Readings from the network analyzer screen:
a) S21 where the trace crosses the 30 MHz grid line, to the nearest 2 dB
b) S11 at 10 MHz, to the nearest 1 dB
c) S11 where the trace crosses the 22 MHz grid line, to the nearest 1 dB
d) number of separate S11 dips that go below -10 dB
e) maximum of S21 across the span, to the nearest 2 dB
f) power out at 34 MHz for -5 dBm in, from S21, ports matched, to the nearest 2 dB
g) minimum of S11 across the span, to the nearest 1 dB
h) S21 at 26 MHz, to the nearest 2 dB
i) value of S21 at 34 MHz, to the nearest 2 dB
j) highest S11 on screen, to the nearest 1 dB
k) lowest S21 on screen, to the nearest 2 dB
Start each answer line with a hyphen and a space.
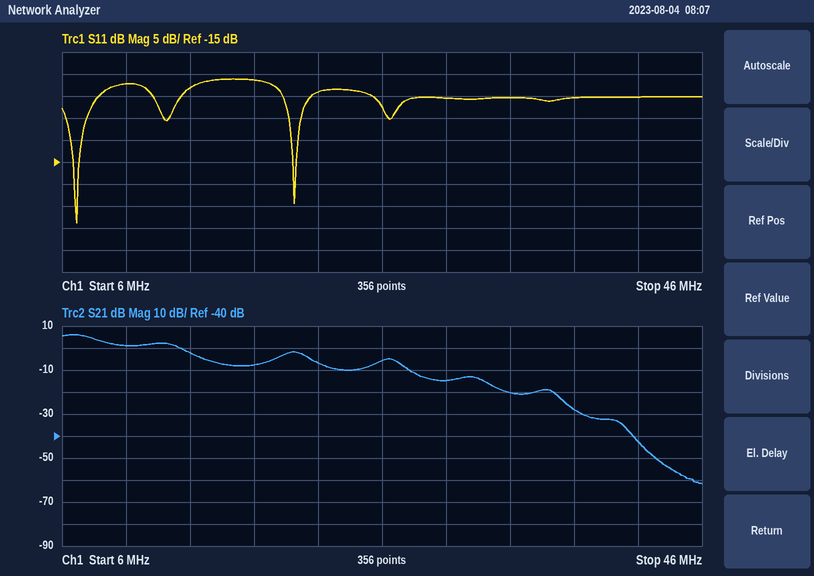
- -14 dB
- 3 dB
- 1 dB
- 2
- 6 dB
- -26 dBm
- -29 dB
- -6 dB
- -20 dB
- 4 dB
- -62 dB
